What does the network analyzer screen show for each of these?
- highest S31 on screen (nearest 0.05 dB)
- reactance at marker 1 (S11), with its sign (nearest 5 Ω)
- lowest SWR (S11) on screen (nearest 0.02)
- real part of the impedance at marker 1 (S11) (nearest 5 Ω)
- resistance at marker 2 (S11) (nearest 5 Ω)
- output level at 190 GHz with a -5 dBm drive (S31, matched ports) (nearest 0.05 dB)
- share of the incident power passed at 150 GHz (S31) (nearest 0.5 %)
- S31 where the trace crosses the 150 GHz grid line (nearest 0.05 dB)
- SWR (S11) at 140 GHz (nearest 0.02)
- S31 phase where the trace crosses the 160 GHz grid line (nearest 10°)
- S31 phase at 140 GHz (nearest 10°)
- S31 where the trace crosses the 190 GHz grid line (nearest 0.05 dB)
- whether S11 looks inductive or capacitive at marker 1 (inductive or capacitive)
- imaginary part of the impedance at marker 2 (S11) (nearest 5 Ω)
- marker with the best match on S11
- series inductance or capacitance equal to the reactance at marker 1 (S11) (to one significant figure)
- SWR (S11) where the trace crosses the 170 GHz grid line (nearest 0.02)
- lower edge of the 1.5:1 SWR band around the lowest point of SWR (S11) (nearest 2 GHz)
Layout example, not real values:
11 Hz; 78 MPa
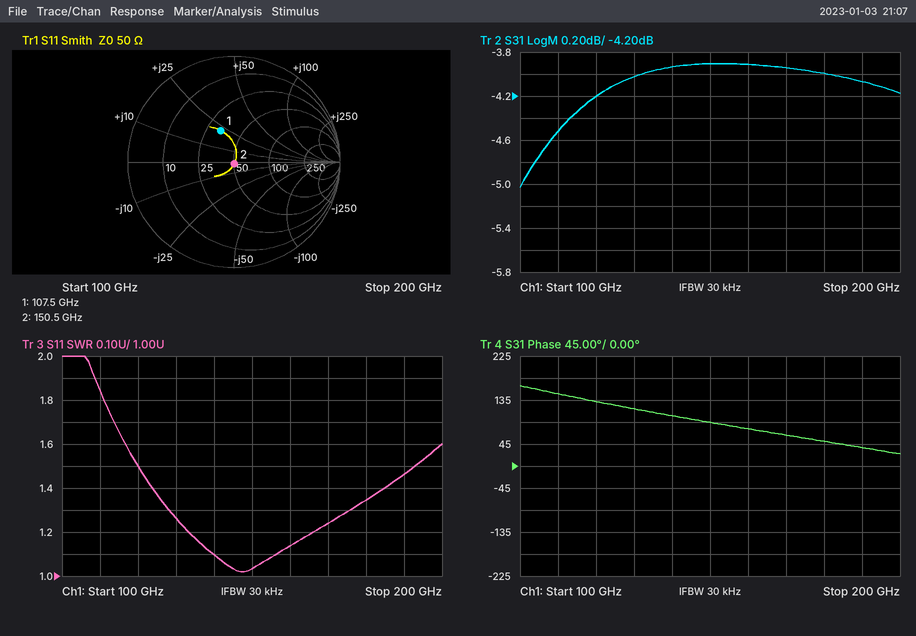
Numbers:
-3.90 dB; +20 Ω; 1.02; 35 Ω; 50 Ω; -9.05 dBm; 40.5 %; -3.90 dB; 1.10; 80°; 100°; -4.05 dB; inductive; 0 Ω; marker 2; 30 pH; 1.24; 120 GHz
